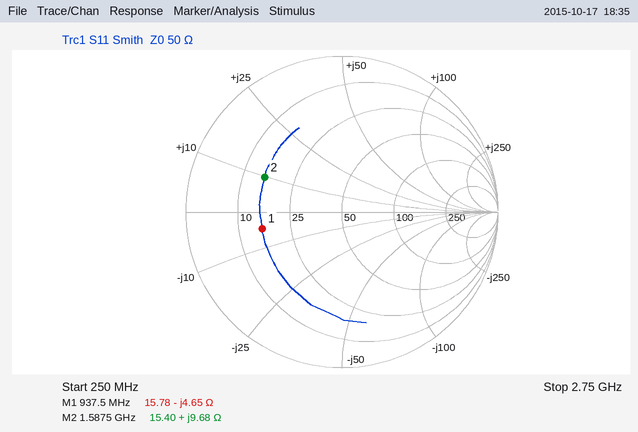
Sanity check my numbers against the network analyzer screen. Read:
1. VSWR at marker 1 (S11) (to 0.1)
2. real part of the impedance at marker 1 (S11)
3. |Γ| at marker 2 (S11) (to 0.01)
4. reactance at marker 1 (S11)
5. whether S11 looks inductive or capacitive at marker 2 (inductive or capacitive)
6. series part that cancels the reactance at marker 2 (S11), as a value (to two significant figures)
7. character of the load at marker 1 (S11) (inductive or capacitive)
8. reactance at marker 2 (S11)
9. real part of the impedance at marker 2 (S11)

3.2
15.78 Ω
0.54
-4.65 Ω
inductive
10 pF
capacitive
+9.68 Ω
15.40 Ω
